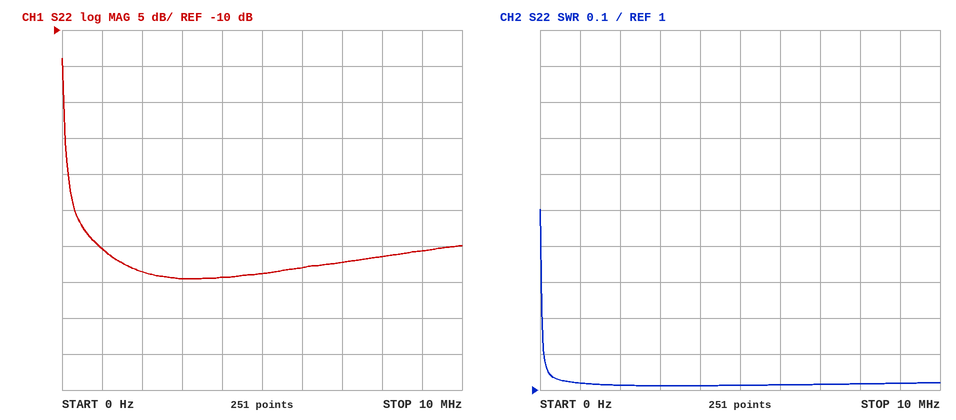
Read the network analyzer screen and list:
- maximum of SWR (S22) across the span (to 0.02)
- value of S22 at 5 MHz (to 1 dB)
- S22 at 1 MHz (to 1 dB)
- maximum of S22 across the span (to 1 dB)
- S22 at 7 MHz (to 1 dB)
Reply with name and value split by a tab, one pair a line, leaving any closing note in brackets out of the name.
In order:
maximum of SWR (S22) across the span	1.50
value of S22 at 5 MHz	-44 dB
S22 at 1 MHz	-40 dB
maximum of S22 across the span	-14 dB
S22 at 7 MHz	-42 dB
